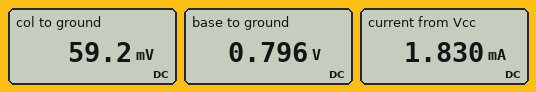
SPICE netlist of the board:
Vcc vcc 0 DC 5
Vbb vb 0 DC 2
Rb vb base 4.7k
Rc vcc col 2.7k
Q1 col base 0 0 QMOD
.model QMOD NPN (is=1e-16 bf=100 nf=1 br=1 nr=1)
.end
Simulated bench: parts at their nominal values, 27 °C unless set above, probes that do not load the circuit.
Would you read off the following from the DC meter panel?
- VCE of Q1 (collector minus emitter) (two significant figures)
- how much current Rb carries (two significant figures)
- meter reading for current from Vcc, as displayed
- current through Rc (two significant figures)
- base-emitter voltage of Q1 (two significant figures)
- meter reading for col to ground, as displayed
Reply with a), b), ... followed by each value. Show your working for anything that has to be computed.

a) 59.2 mV = 59 mV
b) (2 V - 796 mV) / 4.7 kΩ = 260 µA
c) 1.830 mA
d) (5 V - 59.2 mV) / 2.7 kΩ = 1.8 mA
e) 796 mV = 800 mV
f) 59.2 mV
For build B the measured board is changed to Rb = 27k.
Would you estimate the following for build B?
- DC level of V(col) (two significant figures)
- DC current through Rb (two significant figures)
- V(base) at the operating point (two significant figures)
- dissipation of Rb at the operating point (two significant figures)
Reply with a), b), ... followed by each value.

a) 110 mV
b) 45 µA
c) 790 mV
d) 54 µW
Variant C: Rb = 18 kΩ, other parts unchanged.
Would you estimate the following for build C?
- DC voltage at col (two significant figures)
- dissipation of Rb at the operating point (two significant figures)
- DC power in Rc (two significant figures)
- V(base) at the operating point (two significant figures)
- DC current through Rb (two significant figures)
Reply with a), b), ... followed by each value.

a) 95 mV
b) 81 µW
c) 8.9 mW
d) 790 mV
e) 67 µA
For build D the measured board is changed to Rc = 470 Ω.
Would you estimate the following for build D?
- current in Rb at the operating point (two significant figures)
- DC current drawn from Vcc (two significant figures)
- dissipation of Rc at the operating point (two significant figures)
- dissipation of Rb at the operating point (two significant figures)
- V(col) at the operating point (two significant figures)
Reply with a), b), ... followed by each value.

a) 250 µA
b) 10 mA
c) 51 mW
d) 290 µW
e) 110 mV
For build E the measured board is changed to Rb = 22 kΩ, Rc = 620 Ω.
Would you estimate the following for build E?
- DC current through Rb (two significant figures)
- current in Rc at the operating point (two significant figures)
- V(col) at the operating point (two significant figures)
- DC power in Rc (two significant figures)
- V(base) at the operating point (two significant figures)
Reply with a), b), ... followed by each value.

a) 54 µA
b) 5.4 mA
c) 1.7 V
d) 18 mW
e) 820 mV
